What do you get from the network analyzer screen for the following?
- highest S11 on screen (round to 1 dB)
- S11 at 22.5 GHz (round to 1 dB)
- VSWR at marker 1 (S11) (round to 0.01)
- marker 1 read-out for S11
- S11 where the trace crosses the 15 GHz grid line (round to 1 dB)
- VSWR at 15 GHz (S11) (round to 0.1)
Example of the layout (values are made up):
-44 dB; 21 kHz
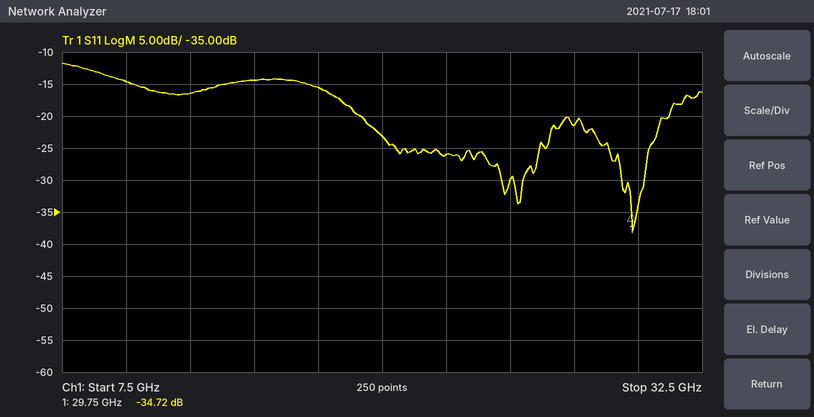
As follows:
-12 dB; -26 dB; 1.04; -34.72 dB; -14 dB; 1.5
